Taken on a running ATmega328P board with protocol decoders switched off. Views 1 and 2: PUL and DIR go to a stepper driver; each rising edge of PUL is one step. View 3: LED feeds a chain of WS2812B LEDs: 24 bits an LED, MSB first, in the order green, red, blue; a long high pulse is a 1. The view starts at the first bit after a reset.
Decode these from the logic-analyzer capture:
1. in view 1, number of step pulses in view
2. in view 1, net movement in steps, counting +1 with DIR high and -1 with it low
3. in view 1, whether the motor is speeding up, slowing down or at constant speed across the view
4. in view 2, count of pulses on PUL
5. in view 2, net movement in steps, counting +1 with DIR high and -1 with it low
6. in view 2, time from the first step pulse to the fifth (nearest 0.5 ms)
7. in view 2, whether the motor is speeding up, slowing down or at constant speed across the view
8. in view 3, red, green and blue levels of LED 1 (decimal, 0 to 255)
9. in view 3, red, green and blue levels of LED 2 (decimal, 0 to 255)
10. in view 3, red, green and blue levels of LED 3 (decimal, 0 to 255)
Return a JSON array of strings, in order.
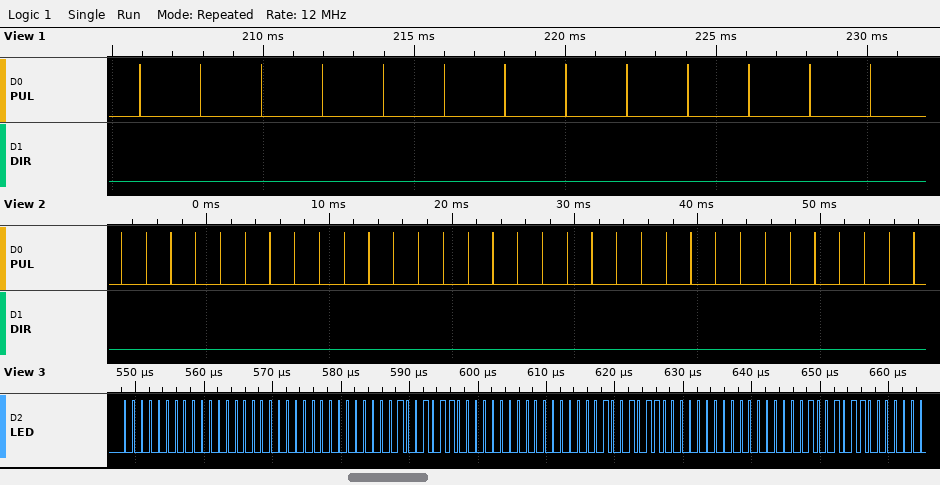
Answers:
["13", "-13", "constant speed", "33", "-33", "8.0 ms", "constant speed", "0, 0, 0", "150, 0, 0", "150, 0, 0"]
